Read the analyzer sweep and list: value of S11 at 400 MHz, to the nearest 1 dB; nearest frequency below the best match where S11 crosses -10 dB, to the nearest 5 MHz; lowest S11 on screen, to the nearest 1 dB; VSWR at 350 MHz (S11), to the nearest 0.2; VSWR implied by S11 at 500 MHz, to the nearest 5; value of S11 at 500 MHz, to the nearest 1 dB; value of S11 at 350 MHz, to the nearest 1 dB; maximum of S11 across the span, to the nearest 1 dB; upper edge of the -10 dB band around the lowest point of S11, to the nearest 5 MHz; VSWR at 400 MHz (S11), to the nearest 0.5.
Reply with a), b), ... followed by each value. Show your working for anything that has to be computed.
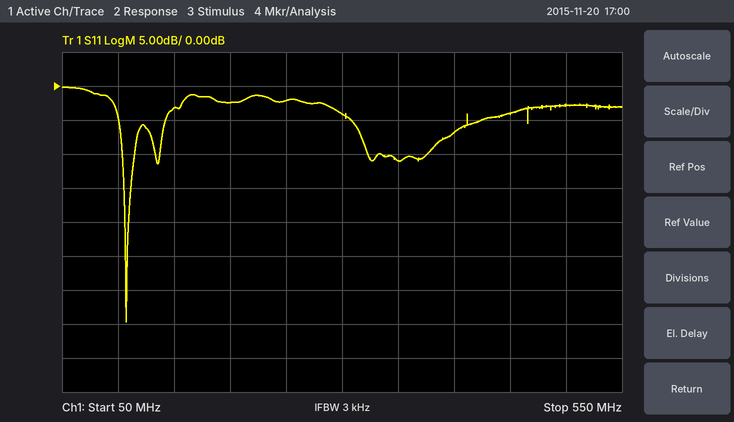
a) -7 dB
b) 105 MHz
c) -35 dB
d) |Γ| = 10^(-11/20) = 0.2818; VSWR = (1 + 0.2818)/(1 − 0.2818) ≈ 1.8
e) |Γ| = 10^(-3/20) = 0.7079; VSWR = (1 + 0.7079)/(1 − 0.7079) ≈ 5.85, so 5 to the nearest 5
f) -3 dB
g) -11 dB
h) 0 dB
i) 115 MHz
j) |Γ| = 10^(-7/20) = 0.4467; VSWR = (1 + 0.4467)/(1 − 0.4467) ≈ 2.61, so 2.5 to the nearest 0.5
